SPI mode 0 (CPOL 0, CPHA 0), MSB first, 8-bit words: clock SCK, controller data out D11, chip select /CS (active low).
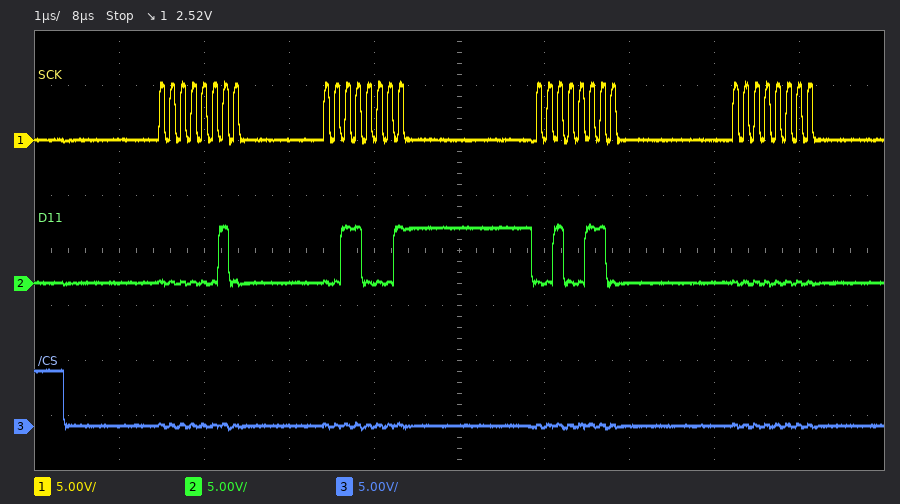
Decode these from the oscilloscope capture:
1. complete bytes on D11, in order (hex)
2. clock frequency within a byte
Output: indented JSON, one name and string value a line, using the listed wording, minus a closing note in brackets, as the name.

{
  "complete bytes on D11, in order": "0x02 0x31 0x26 0x00",
  "clock frequency within a byte": "8 MHz"
}
